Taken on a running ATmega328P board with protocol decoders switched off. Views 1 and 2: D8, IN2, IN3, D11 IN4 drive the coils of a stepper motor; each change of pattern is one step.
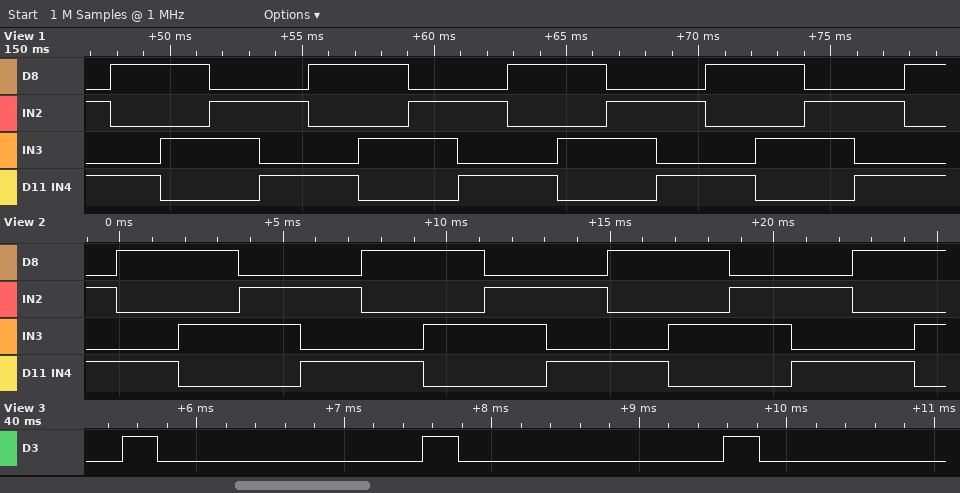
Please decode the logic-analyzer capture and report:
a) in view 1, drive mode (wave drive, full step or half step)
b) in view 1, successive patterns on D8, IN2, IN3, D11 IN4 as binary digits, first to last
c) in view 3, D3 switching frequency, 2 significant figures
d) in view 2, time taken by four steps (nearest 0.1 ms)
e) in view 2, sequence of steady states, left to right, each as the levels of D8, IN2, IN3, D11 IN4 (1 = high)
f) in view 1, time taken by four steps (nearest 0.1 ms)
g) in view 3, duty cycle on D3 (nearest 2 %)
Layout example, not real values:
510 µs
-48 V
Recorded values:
full step
0101 1001 1010 0110 0101 1001 1010 0110 0101 1001 1010 0110 0101 1001 1010 0110 0101 1001
490 Hz
7.5 ms
0101 1001 1010 0110 0101 1001 1010 0110 0101 1001 1010 0110 0101 1001 1010
7.5 ms
12 %
